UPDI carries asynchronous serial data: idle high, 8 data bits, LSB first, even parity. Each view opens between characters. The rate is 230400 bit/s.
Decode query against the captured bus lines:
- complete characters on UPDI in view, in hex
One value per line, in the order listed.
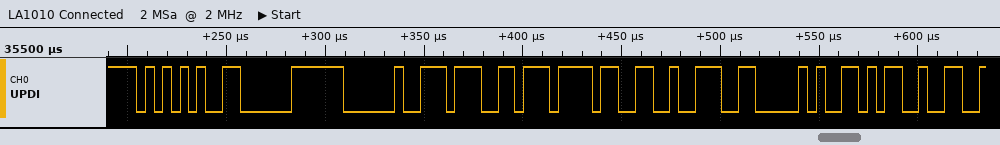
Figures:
55, E0, 20, 67, 6F, 72, 50, 4D
